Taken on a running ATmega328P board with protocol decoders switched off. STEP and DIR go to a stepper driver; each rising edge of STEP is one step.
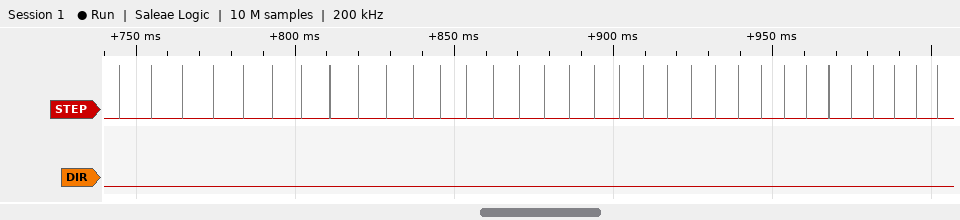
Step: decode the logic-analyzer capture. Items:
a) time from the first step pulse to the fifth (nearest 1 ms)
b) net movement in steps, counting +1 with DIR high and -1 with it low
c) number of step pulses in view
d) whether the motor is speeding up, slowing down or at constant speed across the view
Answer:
39 ms
-33
33
speeding up
